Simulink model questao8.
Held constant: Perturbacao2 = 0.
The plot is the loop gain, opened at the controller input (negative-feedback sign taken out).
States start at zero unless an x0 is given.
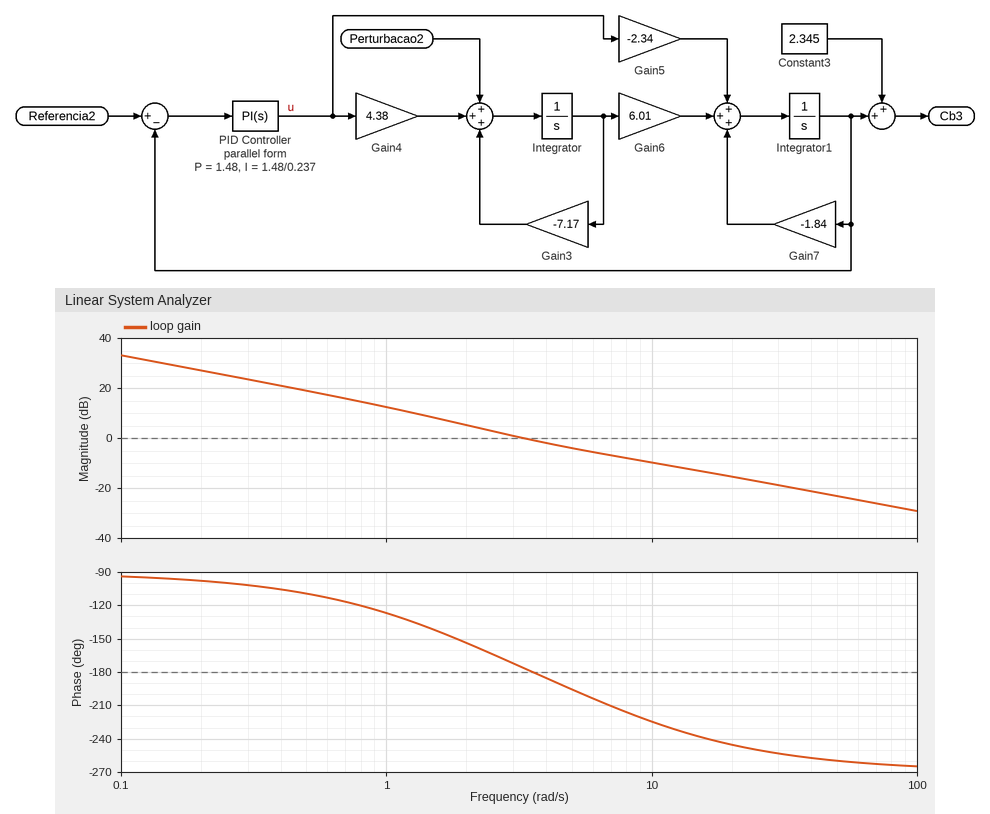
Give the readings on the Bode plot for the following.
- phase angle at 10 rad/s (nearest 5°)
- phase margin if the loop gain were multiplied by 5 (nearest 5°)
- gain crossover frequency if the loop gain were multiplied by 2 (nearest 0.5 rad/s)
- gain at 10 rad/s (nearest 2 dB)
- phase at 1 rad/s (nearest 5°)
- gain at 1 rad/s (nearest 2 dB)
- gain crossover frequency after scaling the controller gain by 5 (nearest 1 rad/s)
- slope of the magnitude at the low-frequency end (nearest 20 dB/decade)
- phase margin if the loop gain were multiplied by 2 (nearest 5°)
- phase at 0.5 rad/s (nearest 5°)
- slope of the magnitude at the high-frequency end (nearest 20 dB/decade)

-225°
-60°
6.5 rad/s
-10 dB
-125°
12 dB
17 rad/s
-20 dB/decade
-25°
-110°
-20 dB/decade
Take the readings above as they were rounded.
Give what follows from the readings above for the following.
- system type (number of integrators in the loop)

1
